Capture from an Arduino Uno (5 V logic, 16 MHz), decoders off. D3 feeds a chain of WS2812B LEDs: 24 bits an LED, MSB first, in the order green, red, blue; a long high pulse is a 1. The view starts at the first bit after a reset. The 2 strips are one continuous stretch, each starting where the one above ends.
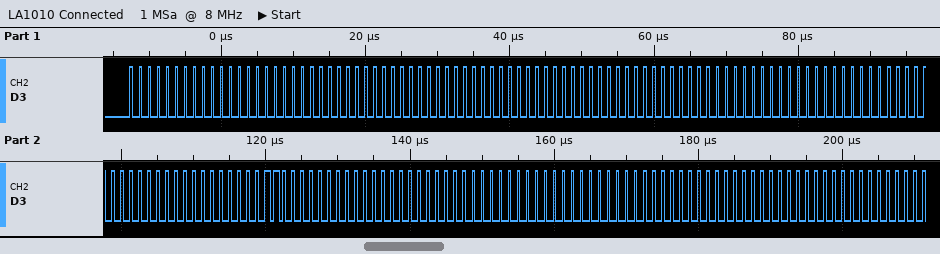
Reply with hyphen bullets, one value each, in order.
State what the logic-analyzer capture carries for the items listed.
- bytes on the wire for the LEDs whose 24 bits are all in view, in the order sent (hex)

- 00 00 00 00 00 00 00 00 00 00 00 00 00 30 00 00 00 00 00 00 00
